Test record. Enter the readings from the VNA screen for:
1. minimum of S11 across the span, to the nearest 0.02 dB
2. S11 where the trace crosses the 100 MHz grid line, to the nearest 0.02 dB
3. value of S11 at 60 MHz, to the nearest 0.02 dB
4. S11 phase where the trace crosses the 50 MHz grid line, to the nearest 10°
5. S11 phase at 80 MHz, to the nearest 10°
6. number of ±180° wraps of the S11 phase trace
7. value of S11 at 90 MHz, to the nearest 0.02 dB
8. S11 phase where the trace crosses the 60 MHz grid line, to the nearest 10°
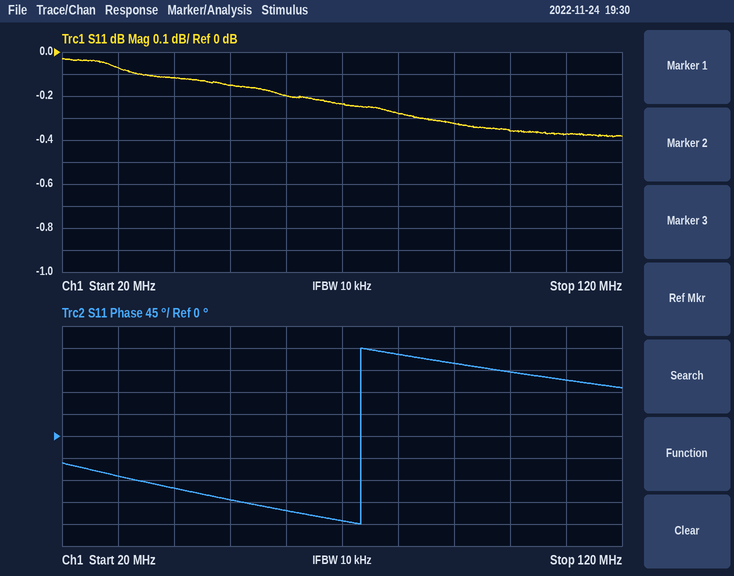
-0.38 dB
-0.36 dB
-0.20 dB
-130°
170°
1
-0.32 dB
-150°
